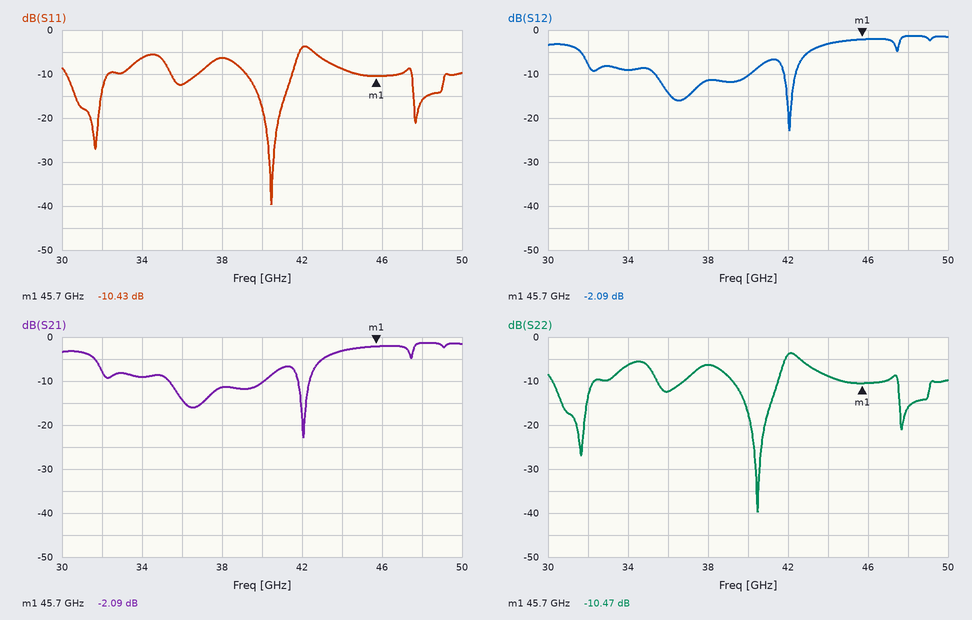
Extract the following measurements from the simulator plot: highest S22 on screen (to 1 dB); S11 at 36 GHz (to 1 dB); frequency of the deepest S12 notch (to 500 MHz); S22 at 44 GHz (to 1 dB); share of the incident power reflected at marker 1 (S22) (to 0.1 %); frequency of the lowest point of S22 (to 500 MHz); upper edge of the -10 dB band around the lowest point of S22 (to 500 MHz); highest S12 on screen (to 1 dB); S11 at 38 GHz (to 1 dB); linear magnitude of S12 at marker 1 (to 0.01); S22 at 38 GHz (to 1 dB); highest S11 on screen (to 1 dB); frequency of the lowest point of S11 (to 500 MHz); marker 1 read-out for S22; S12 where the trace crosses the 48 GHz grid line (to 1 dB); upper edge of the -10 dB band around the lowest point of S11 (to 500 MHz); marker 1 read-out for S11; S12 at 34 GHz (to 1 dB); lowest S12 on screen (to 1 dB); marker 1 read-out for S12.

-4 dB
-12 dB
42.0 GHz
-9 dB
9.0 %
40.5 GHz
41.5 GHz
-1 dB
-6 dB
0.79
-6 dB
-4 dB
40.5 GHz
-10.47 dB
-1 dB
41.5 GHz
-10.43 dB
-9 dB
-23 dB
-2.09 dB
